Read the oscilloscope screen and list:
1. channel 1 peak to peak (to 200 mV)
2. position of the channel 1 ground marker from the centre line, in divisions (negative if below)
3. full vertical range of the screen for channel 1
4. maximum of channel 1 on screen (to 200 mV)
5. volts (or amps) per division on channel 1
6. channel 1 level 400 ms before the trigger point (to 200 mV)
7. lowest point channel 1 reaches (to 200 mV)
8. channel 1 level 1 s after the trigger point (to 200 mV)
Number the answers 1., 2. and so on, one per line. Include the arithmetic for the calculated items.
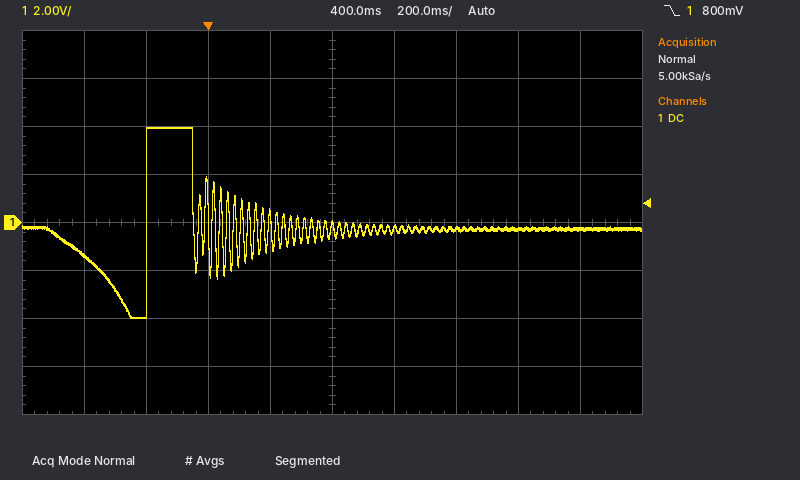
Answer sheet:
1. 4.0 V − (-4.0 V) = 8.0 V
2. 0.0 div
3. 16 V
4. 4.0 V
5. 2 V
6. -1.4 V
7. -4.0 V
8. -200 mV
